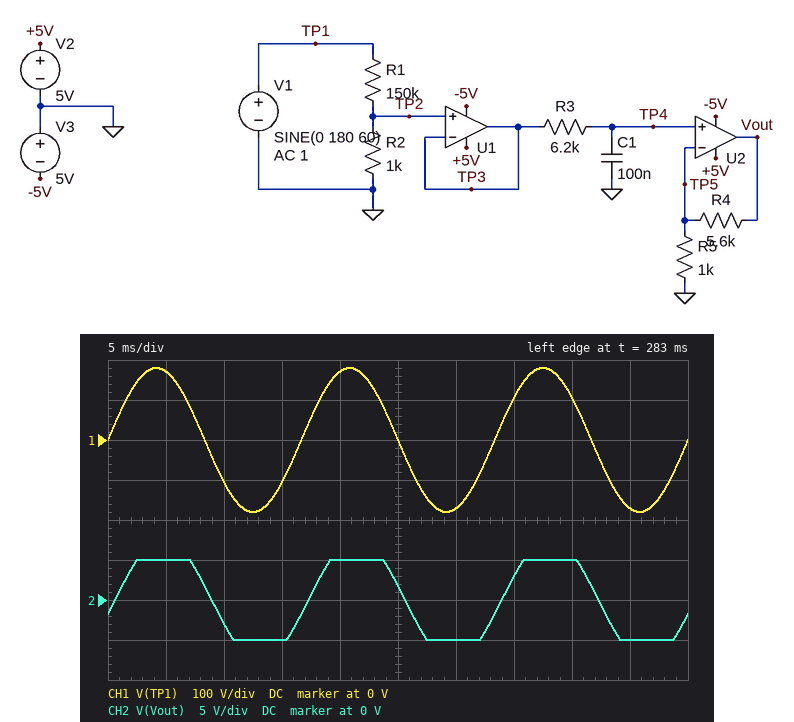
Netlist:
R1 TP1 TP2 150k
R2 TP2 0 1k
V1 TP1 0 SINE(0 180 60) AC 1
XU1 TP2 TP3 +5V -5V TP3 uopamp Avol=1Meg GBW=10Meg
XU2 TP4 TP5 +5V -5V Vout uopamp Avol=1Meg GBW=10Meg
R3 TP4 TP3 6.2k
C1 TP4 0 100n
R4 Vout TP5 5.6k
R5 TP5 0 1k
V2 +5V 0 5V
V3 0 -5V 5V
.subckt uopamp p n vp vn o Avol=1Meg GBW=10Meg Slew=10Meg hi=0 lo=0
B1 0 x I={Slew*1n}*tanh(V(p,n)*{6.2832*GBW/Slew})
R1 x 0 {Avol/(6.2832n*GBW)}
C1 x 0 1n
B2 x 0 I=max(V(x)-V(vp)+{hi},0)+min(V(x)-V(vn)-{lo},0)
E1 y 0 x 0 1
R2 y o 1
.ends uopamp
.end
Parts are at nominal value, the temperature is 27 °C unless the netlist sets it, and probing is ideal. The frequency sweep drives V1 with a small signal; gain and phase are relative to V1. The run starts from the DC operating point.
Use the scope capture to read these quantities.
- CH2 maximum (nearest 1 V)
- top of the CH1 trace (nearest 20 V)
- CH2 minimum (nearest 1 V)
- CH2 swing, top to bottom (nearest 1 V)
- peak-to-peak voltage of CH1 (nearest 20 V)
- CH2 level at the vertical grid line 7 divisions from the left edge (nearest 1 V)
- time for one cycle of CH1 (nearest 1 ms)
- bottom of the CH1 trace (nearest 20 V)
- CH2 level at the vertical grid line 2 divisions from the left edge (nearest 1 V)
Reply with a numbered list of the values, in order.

1. 5 V
2. 180 V
3. -5 V
4. 10 V
5. 360 V
6. 3 V
7. 17 ms
8. -180 V
9. -3 V
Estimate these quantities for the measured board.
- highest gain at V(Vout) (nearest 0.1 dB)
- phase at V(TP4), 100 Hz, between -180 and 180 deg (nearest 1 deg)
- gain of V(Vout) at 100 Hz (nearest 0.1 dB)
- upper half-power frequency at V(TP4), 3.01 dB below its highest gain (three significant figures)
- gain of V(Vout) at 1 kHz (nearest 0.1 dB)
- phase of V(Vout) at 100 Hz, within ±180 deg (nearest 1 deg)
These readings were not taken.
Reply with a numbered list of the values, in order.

1. -27.2 dB
2. -21 deg
3. -27.8 dB
4. 257 Hz
5. -39.3 dB
6. -21 deg
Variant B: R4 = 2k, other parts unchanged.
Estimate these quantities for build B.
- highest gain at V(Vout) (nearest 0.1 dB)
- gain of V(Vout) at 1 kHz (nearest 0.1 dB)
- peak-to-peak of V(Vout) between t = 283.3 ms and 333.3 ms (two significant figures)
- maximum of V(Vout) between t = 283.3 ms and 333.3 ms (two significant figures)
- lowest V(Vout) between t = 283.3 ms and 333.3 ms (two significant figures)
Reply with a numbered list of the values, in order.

1. -34.0 dB
2. -46.1 dB
3. 7.0 V
4. 3.5 V
5. -3.5 V
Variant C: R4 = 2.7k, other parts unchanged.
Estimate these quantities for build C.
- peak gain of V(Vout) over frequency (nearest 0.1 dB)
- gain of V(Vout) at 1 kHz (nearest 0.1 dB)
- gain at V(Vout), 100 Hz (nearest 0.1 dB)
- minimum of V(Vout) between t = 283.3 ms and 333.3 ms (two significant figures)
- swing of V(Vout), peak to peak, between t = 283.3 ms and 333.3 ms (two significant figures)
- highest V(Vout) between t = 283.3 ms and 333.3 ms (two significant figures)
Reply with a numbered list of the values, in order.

1. -32.2 dB
2. -44.3 dB
3. -32.8 dB
4. -4.3 V
5. 8.6 V
6. 4.3 V
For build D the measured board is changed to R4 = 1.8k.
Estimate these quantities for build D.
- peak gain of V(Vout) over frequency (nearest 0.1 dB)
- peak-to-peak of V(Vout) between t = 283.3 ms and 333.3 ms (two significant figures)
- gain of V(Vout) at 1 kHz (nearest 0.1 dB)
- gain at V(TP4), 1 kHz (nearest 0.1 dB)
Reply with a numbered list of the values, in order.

1. -34.6 dB
2. 6.5 V
3. -46.7 dB
4. -55.7 dB
